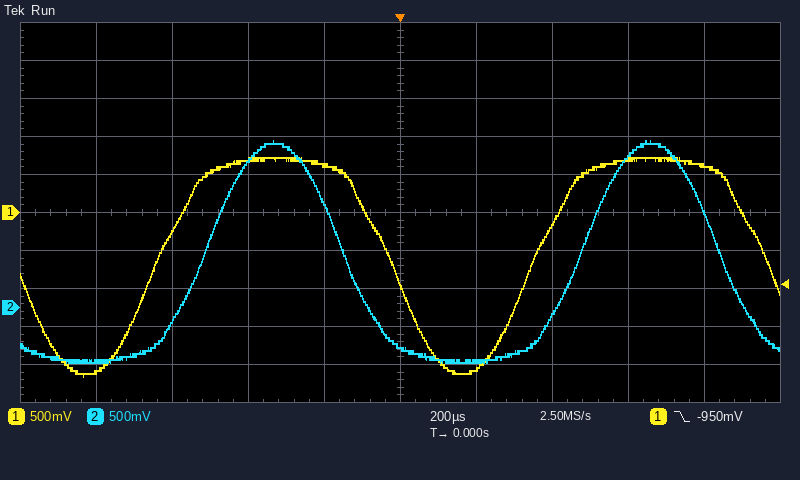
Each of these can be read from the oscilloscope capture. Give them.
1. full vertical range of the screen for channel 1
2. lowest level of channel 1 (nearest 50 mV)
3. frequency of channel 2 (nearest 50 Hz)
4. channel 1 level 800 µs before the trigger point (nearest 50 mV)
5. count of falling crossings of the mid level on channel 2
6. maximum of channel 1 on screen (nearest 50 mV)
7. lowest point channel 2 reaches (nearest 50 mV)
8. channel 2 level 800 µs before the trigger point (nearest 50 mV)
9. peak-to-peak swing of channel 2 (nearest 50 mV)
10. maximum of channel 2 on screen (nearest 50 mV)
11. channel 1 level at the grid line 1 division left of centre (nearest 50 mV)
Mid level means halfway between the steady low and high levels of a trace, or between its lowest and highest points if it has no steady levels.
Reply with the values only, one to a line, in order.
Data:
5 V
-2.15 V
1.00 kHz
-2.10 V
2
700 mV
-700 mV
-700 mV
2.90 V
2.20 V
600 mV
